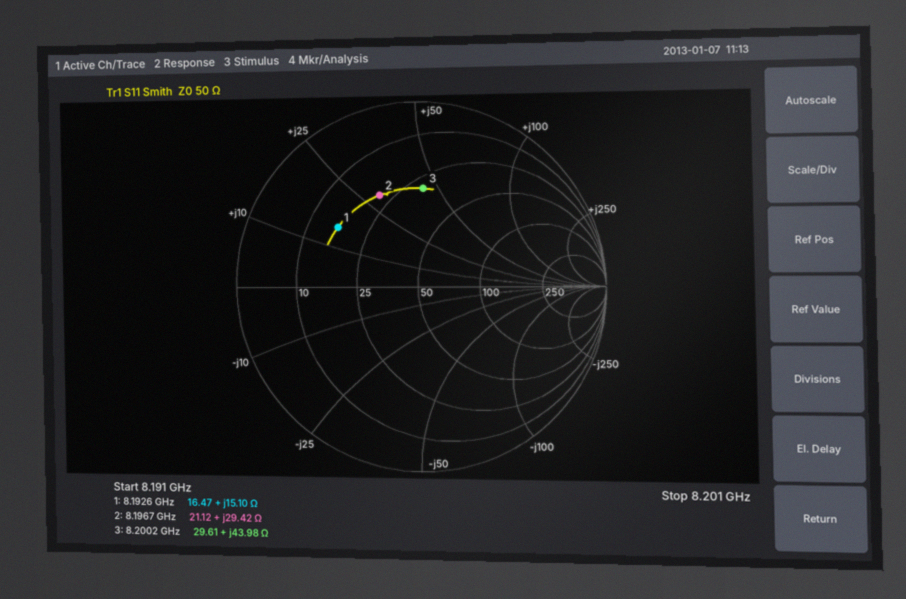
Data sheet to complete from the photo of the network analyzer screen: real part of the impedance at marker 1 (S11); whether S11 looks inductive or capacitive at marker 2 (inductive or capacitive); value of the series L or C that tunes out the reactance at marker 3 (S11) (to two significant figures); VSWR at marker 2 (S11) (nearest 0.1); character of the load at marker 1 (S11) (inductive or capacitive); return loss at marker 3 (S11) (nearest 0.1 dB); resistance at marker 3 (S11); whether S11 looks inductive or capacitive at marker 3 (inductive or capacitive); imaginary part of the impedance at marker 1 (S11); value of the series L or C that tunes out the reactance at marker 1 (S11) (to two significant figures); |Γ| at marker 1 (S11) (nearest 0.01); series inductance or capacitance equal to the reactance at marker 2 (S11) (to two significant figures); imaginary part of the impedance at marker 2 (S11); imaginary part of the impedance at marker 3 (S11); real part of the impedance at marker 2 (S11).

16.47 Ω
inductive
440 fF
3.3
inductive
5.5 dB
29.61 Ω
inductive
+15.10 Ω
1.3 pF
0.54
570 pH
+29.42 Ω
+43.98 Ω
21.12 Ω
